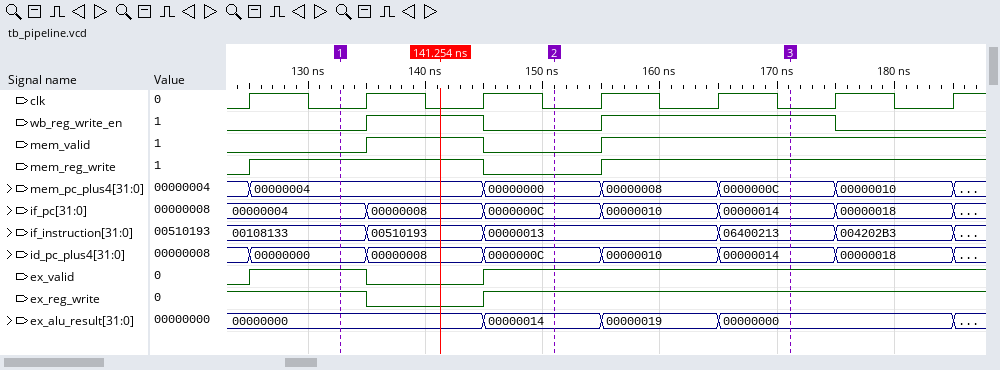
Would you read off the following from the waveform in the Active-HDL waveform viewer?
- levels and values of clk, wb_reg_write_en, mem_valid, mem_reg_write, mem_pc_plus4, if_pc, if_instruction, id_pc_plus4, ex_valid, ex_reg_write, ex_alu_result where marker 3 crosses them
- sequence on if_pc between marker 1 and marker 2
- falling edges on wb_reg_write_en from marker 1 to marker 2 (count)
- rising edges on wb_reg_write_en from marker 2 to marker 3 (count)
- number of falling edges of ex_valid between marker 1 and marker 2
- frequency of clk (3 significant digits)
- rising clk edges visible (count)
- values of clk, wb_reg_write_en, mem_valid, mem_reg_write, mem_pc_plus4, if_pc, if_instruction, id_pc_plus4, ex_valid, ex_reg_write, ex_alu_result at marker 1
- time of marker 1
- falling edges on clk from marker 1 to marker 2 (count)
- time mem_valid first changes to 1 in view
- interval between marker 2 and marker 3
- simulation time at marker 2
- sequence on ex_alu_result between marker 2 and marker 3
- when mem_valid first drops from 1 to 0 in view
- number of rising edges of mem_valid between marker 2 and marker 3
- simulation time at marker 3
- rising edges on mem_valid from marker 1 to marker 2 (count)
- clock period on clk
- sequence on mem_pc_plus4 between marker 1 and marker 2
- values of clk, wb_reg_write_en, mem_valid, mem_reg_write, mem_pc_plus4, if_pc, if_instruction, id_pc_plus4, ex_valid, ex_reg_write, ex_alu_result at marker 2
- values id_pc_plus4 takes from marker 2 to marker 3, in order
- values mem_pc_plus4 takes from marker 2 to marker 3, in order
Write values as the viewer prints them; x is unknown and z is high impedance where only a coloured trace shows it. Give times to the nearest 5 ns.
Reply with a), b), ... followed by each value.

a) clk=0, wb_reg_write_en=1, mem_valid=1, mem_reg_write=1, mem_pc_plus4=0000000C, if_pc=00000014, if_instruction=06400213, id_pc_plus4=00000014, ex_valid=1, ex_reg_write=1, ex_alu_result=00000000
b) 00000004, 00000008, 0000000C
c) 1
d) 1
e) 1
f) 100 MHz
g) 7
h) clk=0, wb_reg_write_en=0, mem_valid=0, mem_reg_write=1, mem_pc_plus4=00000004, if_pc=00000004, if_instruction=00108133, id_pc_plus4=00000000, ex_valid=1, ex_reg_write=1, ex_alu_result=00000000
i) 135 ns
j) 2
k) 135 ns
l) 20 ns
m) 150 ns
n) 00000014, 00000019, 00000000
o) 145 ns
p) 1
q) 170 ns
r) 1
s) 10 ns
t) 00000004, 00000000
u) clk=0, wb_reg_write_en=0, mem_valid=0, mem_reg_write=0, mem_pc_plus4=00000000, if_pc=0000000C, if_instruction=00000013, id_pc_plus4=0000000C, ex_valid=1, ex_reg_write=1, ex_alu_result=00000014
v) 0000000C, 00000010, 00000014
w) 00000000, 00000008, 0000000C
